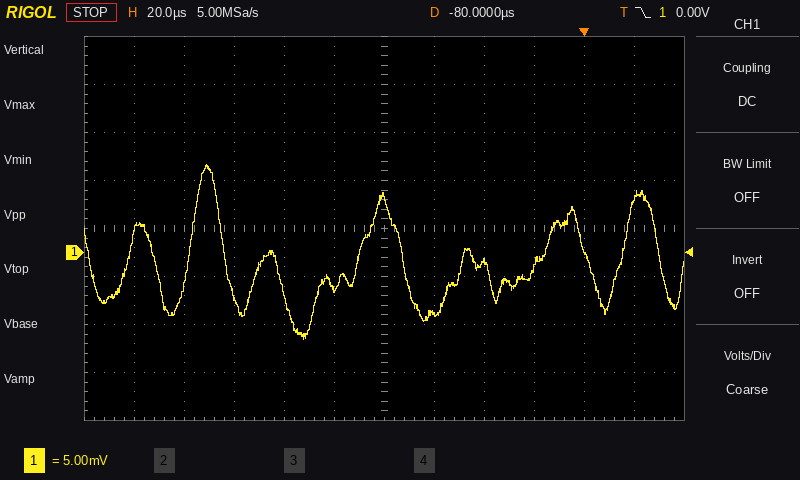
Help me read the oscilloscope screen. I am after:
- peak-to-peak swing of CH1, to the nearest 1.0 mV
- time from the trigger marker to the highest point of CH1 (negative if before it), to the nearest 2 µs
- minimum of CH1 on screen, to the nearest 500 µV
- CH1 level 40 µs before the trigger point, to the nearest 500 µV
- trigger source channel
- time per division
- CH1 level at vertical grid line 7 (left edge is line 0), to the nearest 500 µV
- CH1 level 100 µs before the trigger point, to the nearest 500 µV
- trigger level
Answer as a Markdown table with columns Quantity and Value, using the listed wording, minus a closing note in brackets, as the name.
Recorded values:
| Quantity | Value |
|---|---|
| peak-to-peak swing of CH1, to the nearest 1.0 mV | 18.0 mV |
| time from the trigger marker to the highest point of CH1 (negative if before it), to the nearest 2 µs | -150 µs |
| minimum of CH1 on screen, to the nearest 500 µV | -9.0 mV |
| CH1 level 40 µs before the trigger point, to the nearest 500 µV | -1.0 mV |
| trigger source channel | CH1 |
| time per division | 20 µs |
| CH1 level at vertical grid line 7 (left edge is line 0), to the nearest 500 µV | -6.5 mV |
| CH1 level 100 µs before the trigger point, to the nearest 500 µV | -4.0 mV |
| trigger level | 0.00 V |
